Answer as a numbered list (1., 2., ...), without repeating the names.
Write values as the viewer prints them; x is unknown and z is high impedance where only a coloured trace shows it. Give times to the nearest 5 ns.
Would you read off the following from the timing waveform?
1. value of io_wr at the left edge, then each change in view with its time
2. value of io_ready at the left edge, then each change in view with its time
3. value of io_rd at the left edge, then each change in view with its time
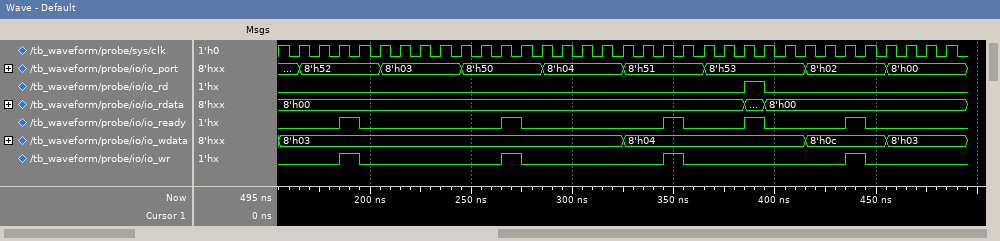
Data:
1. 0, 1 at 185 ns, 0 at 195 ns, 1 at 265 ns, 0 at 275 ns, 1 at 345 ns, 0 at 355 ns, 1 at 435 ns, 0 at 445 ns
2. 0, 1 at 185 ns, 0 at 195 ns, 1 at 265 ns, 0 at 275 ns, 1 at 345 ns, 0 at 355 ns, 1 at 385 ns, 0 at 395 ns, 1 at 435 ns, 0 at 445 ns
3. 0, 1 at 385 ns, 0 at 395 ns
